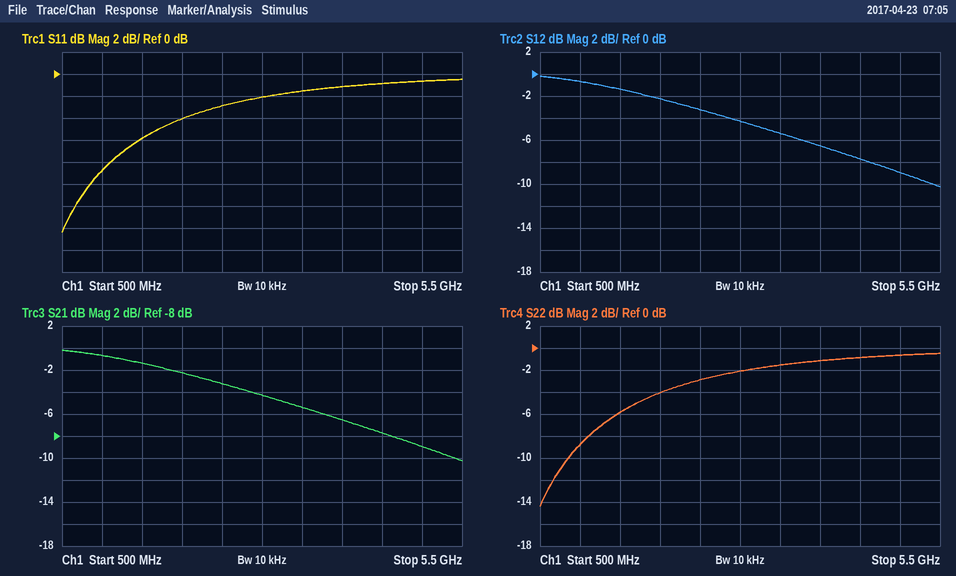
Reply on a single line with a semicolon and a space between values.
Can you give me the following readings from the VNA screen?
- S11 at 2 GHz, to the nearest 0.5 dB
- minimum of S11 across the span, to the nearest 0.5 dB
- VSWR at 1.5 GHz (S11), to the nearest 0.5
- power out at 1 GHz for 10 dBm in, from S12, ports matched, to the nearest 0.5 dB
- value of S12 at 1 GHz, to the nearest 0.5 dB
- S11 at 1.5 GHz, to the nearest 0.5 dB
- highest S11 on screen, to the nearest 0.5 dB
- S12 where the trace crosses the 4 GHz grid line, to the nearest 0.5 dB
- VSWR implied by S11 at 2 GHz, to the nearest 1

-4.0 dB; -14.5 dB; 3.0; 9.5 dBm; -0.5 dB; -6.0 dB; -0.5 dB; -6.5 dB; 4
